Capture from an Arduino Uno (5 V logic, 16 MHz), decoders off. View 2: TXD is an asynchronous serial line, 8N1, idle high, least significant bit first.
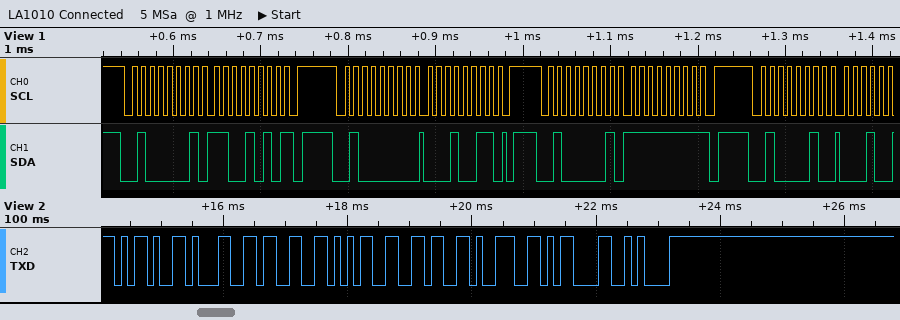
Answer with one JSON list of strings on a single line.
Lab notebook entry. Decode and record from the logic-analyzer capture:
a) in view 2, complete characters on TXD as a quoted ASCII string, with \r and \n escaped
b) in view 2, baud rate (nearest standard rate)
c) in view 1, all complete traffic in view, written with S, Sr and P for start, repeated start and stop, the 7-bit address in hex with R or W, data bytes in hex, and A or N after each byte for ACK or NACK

["\"-13569\\r\\n\"", "9600 baud", "S 20R A CA N P S 20W A 13 A P S 20R A FF N P S 21W A"]
